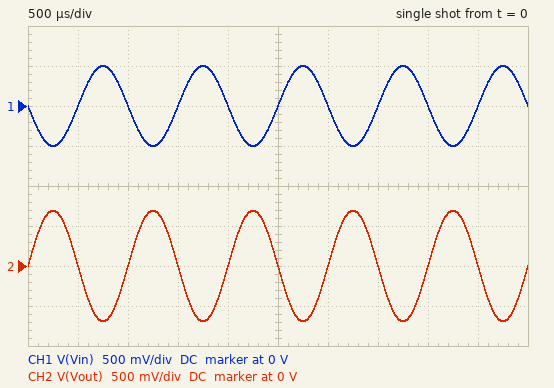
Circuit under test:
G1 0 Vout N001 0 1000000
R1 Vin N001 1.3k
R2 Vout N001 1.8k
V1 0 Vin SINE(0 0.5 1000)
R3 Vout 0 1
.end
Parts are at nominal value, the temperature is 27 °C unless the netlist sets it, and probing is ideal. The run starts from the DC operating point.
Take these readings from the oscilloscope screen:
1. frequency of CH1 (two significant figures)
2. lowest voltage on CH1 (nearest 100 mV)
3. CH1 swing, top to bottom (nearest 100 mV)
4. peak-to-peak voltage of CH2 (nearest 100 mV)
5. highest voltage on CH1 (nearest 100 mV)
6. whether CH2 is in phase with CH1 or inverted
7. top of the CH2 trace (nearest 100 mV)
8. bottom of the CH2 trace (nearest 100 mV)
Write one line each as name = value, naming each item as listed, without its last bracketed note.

frequency of CH1 = 1.0 kHz
lowest voltage on CH1 = -500 mV
CH1 swing, top to bottom = 1.0 V
peak-to-peak voltage of CH2 = 1.4 V
highest voltage on CH1 = 500 mV
whether CH2 is in phase with CH1 or inverted = inverted
top of the CH2 trace = 700 mV
bottom of the CH2 trace = -700 mV
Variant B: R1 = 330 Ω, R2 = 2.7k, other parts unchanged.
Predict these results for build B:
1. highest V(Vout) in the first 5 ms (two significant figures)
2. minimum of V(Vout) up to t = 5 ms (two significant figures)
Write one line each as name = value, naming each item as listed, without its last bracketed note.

highest V(Vout) in the first 5 ms = 4.1 V
minimum of V(Vout) up to t = 5 ms = -4.1 V
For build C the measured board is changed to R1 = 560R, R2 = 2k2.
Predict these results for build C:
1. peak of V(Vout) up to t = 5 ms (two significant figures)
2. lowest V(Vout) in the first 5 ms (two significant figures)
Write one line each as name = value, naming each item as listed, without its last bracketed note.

peak of V(Vout) up to t = 5 ms = 2.0 V
lowest V(Vout) in the first 5 ms = -2.0 V
